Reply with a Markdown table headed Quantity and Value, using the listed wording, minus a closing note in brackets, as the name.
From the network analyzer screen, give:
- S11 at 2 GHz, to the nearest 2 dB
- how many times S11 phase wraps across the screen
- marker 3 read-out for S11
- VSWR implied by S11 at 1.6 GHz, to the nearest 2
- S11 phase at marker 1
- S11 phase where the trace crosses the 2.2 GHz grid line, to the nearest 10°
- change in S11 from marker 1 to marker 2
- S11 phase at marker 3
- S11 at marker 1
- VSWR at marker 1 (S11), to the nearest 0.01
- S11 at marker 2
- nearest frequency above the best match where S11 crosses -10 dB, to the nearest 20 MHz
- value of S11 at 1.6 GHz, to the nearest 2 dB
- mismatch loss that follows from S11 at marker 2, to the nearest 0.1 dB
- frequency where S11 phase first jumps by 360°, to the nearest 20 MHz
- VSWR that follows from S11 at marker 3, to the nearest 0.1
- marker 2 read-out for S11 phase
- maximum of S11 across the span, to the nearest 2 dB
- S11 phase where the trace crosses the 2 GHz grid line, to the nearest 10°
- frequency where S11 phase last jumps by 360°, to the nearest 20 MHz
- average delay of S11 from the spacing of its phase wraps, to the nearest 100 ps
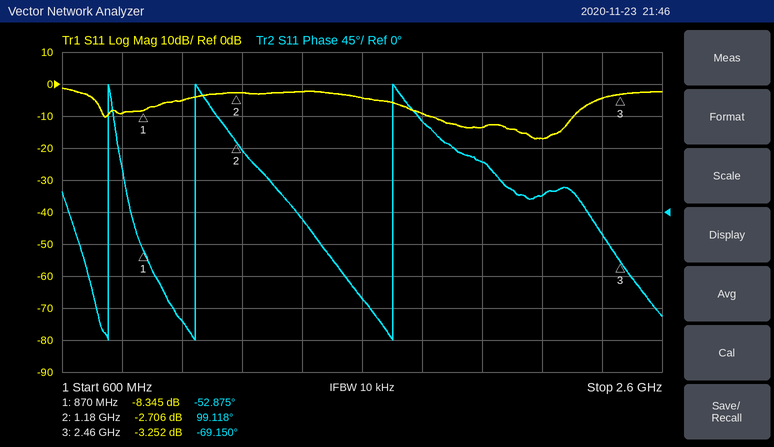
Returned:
| Quantity | Value |
|---|---|
| S11 at 2 GHz, to the nearest 2 dB | -14 dB |
| how many times S11 phase wraps across the screen | 3 |
| marker 3 read-out for S11 | -3.252 dB |
| VSWR implied by S11 at 1.6 GHz, to the nearest 2 | 4 |
| S11 phase at marker 1 | -52.875° |
| S11 phase where the trace crosses the 2.2 GHz grid line, to the nearest 10° | 20° |
| change in S11 from marker 1 to marker 2 | 5.639 dB |
| S11 phase at marker 3 | -69.150° |
| S11 at marker 1 | -8.345 dB |
| VSWR at marker 1 (S11), to the nearest 0.01 | 2.24 |
| S11 at marker 2 | -2.706 dB |
| nearest frequency above the best match where S11 crosses -10 dB, to the nearest 20 MHz | 2.30 GHz |
| value of S11 at 1.6 GHz, to the nearest 2 dB | -4 dB |
| mismatch loss that follows from S11 at marker 2, to the nearest 0.1 dB | 3.3 dB |
| frequency where S11 phase first jumps by 360°, to the nearest 20 MHz | 760 MHz |
| VSWR that follows from S11 at marker 3, to the nearest 0.1 | 5.4 |
| marker 2 read-out for S11 phase | 99.118° |
| maximum of S11 across the span, to the nearest 2 dB | -2 dB |
| S11 phase where the trace crosses the 2 GHz grid line, to the nearest 10° | 70° |
| frequency where S11 phase last jumps by 360°, to the nearest 20 MHz | 1.70 GHz |
| average delay of S11 from the spacing of its phase wraps, to the nearest 100 ps | 2.1 ns |
